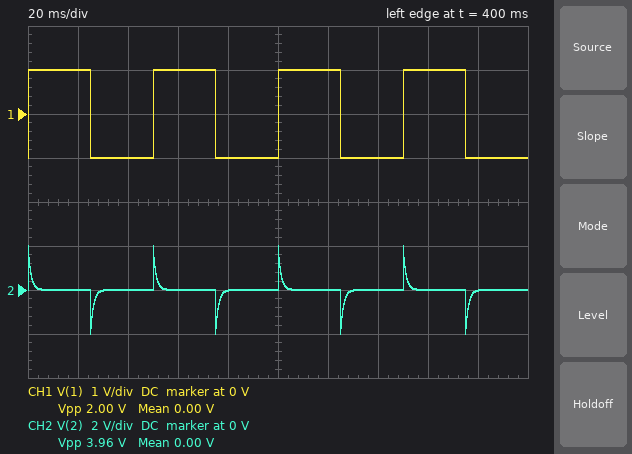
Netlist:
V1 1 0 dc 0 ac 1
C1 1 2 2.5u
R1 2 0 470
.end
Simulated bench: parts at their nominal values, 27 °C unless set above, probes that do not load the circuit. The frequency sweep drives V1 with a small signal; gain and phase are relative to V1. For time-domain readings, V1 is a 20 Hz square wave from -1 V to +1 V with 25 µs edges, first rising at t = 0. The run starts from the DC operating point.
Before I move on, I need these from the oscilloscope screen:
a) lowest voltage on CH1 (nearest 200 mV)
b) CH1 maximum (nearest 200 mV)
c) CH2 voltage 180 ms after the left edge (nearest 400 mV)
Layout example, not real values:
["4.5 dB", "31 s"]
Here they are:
["-1.0 V", "1.0 V", "0 V"]
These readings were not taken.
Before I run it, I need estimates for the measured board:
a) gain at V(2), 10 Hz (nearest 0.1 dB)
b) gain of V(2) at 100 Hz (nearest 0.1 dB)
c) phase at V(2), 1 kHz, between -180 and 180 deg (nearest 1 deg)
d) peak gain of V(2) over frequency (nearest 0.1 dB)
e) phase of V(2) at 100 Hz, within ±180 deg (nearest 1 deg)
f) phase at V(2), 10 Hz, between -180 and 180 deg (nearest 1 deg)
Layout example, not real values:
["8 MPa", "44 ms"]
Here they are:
["-22.7 dB", "-4.5 dB", "8 deg", "0 dB", "54 deg", "86 deg"]
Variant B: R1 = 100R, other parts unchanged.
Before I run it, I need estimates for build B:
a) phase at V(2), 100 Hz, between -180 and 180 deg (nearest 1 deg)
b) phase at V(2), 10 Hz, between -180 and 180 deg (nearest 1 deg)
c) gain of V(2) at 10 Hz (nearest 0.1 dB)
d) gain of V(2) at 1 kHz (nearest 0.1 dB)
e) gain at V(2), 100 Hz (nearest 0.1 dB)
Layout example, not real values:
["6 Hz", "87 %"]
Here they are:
["81 deg", "89 deg", "-36.1 dB", "-1.5 dB", "-16.2 dB"]
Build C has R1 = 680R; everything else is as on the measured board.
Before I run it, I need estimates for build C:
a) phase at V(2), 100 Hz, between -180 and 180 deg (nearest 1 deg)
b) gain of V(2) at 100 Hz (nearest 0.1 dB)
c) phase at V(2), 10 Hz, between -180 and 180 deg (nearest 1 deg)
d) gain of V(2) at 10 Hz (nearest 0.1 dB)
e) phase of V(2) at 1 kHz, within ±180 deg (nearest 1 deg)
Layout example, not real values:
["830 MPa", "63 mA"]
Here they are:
["43 deg", "-2.7 dB", "84 deg", "-19.5 dB", "5 deg"]
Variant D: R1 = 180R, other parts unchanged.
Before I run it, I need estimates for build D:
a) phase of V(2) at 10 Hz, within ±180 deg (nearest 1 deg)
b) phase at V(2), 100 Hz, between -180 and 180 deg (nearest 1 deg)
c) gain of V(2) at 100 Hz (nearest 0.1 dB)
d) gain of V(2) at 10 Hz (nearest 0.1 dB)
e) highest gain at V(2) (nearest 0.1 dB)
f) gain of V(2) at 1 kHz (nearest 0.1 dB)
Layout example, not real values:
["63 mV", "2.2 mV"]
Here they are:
["88 deg", "74 deg", "-11.3 dB", "-31.0 dB", "0 dB", "-0.5 dB"]
